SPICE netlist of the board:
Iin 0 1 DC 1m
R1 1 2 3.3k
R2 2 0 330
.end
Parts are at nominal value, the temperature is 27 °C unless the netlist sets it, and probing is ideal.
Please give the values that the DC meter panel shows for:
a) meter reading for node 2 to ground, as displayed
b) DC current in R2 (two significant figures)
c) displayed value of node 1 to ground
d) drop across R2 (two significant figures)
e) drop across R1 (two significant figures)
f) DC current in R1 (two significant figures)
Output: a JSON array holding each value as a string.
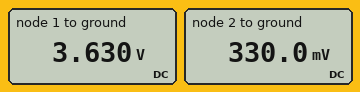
["330.0 mV", "1.0 mA", "3.630 V", "330 mV", "3.3 V", "1.0 mA"]
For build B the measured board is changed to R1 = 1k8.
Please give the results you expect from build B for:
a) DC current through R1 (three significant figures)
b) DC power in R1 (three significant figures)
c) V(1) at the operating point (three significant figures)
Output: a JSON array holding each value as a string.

["1.00 mA", "1.80 mW", "2.13 V"]
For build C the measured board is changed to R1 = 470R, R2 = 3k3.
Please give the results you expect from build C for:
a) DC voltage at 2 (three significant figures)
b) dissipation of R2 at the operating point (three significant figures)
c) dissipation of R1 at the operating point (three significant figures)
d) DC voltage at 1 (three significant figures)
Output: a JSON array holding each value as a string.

["3.30 V", "3.30 mW", "470 µW", "3.77 V"]
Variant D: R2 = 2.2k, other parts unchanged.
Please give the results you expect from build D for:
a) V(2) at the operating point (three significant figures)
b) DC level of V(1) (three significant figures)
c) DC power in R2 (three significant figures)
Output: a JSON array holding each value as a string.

["2.20 V", "5.50 V", "2.20 mW"]
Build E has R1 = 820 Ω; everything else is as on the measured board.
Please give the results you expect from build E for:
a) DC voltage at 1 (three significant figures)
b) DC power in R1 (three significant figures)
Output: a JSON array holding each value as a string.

["1.15 V", "820 µW"]
